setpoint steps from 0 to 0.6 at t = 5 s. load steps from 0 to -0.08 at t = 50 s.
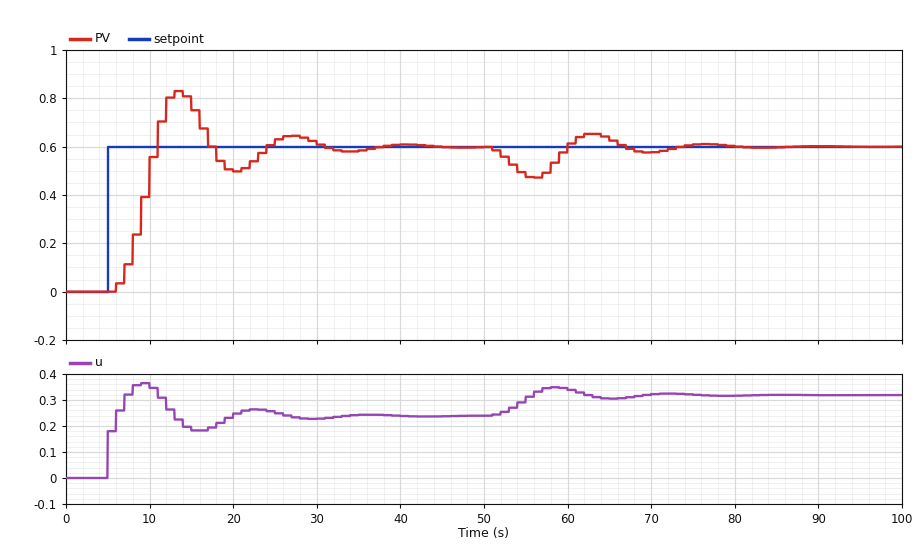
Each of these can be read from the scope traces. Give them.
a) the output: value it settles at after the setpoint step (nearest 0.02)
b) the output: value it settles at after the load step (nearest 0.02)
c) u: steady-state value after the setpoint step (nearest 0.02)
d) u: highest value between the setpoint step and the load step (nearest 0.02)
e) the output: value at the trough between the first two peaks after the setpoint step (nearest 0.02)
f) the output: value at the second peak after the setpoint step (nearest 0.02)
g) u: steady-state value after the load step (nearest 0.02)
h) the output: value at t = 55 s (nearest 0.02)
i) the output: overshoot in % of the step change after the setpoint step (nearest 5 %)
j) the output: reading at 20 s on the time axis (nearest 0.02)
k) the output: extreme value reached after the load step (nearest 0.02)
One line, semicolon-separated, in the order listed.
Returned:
0.60; 0.60; 0.24; 0.36; 0.50; 0.64; 0.32; 0.48; 40 %; 0.50; 0.48
